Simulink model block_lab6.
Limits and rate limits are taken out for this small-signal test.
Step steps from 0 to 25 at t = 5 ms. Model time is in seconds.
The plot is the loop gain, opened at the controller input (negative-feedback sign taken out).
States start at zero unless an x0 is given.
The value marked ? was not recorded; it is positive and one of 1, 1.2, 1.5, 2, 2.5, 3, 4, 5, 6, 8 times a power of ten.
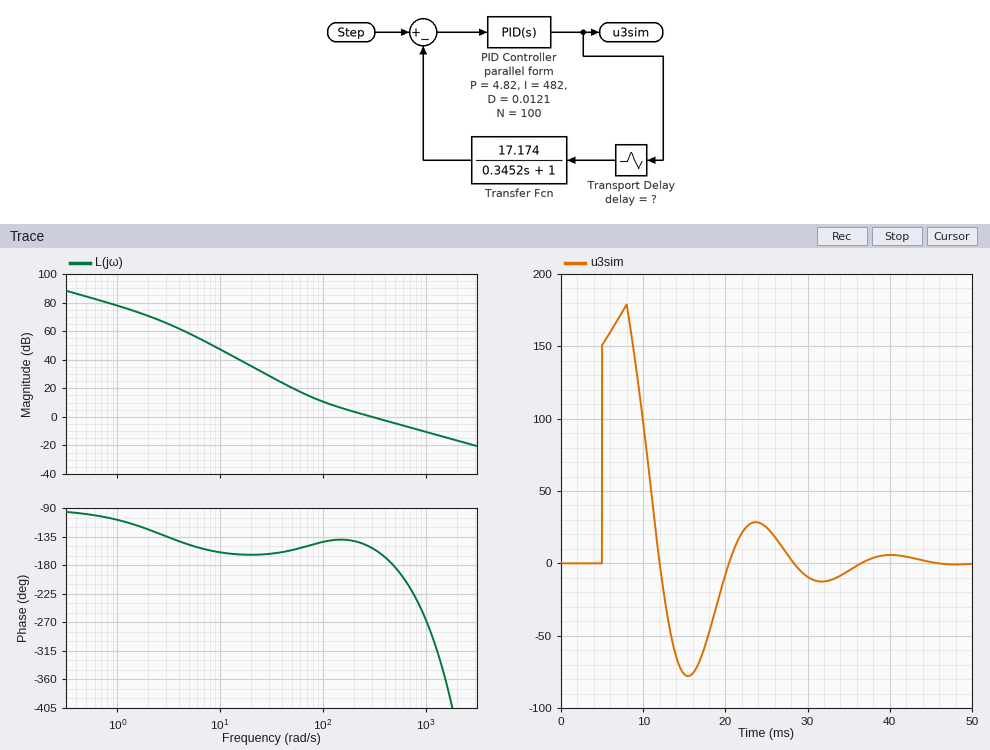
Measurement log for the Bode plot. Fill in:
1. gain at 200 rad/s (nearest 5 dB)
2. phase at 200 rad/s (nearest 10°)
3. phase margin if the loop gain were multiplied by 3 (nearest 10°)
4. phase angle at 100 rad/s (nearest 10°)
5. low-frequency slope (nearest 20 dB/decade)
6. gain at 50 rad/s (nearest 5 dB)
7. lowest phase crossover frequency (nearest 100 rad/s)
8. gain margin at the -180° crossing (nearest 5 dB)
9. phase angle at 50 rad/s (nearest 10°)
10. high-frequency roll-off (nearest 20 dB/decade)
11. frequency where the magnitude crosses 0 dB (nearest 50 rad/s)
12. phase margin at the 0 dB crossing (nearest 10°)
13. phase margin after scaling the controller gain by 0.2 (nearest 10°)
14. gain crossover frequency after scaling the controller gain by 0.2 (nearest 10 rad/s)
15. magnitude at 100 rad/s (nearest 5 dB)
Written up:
5 dB
-140°
-70°
-140°
-20 dB/decade
20 dB
500 rad/s
5 dB
-160°
-20 dB/decade
300 rad/s
30°
30°
80 rad/s
10 dB
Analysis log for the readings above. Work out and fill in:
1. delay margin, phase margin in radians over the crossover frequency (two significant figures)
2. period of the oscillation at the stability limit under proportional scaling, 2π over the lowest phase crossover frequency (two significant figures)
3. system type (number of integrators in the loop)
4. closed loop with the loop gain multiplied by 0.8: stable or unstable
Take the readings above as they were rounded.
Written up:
0.0017 s
0.013 s
1
stable
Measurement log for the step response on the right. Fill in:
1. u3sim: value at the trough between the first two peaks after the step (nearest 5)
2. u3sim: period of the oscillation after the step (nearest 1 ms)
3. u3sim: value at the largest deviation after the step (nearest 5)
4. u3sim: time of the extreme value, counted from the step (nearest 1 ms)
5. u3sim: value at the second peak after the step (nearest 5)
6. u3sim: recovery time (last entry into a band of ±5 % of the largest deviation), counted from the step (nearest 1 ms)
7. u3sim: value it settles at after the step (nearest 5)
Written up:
-80
16 ms
180
3 ms
30
29 ms
0
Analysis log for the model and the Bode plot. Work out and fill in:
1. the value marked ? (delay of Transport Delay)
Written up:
0.003
